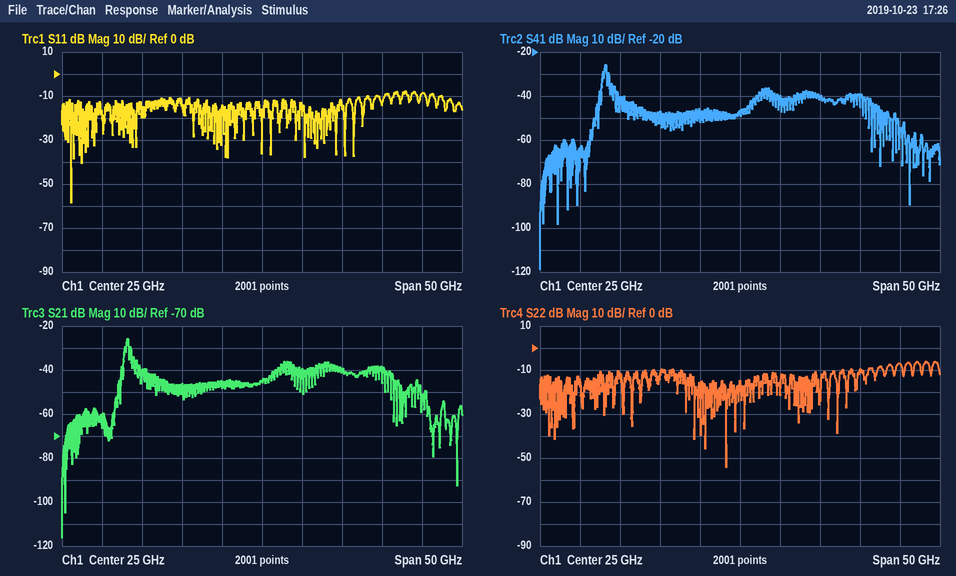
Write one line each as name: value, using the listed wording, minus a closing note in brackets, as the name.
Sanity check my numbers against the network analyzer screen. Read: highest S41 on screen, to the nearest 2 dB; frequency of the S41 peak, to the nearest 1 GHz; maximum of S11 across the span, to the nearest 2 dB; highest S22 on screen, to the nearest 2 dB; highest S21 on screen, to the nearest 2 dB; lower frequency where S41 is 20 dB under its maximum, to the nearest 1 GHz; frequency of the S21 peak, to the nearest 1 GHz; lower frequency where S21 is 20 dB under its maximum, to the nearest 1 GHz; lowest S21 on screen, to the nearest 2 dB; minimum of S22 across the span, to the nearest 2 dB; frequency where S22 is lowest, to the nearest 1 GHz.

highest S41 on screen, to the nearest 2 dB: -26 dB
frequency of the S41 peak, to the nearest 1 GHz: 8 GHz
maximum of S11 across the span, to the nearest 2 dB: -8 dB
highest S22 on screen, to the nearest 2 dB: -6 dB
highest S21 on screen, to the nearest 2 dB: -26 dB
lower frequency where S41 is 20 dB under its maximum, to the nearest 1 GHz: 7 GHz
frequency of the S21 peak, to the nearest 1 GHz: 8 GHz
lower frequency where S21 is 20 dB under its maximum, to the nearest 1 GHz: 7 GHz
lowest S21 on screen, to the nearest 2 dB: -116 dB
minimum of S22 across the span, to the nearest 2 dB: -54 dB
frequency where S22 is lowest, to the nearest 1 GHz: 23 GHz
